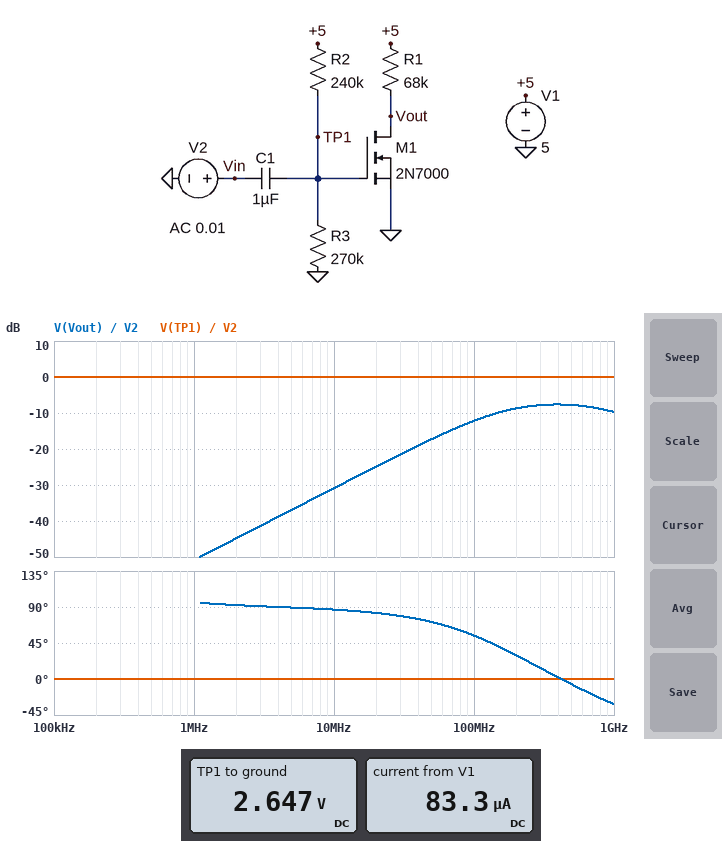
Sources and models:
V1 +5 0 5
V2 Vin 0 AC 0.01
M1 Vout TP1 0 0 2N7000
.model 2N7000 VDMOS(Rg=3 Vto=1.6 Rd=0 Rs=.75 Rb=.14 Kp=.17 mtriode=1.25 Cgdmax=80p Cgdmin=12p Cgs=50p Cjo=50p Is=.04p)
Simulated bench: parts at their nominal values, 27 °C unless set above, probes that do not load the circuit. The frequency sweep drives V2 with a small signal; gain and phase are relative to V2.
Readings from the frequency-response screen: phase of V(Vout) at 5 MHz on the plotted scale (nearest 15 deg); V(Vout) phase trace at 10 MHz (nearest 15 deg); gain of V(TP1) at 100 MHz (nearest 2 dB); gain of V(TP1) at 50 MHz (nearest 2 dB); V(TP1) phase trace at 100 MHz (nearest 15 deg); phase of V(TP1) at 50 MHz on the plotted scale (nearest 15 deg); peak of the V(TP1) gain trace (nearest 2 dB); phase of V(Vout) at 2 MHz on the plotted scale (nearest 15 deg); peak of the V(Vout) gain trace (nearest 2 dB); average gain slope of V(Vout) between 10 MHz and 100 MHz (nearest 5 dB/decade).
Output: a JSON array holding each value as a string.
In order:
["90 deg", "90 deg", "0 dB", "0 dB", "0 deg", "0 deg", "0 dB", "90 deg", "-8 dB", "20 dB/decade"]
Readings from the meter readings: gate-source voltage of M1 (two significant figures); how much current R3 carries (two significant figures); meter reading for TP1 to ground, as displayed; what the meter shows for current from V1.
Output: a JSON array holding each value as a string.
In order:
["2.6 V", "9.8 µA", "2.647 V", "83.3 µA"]
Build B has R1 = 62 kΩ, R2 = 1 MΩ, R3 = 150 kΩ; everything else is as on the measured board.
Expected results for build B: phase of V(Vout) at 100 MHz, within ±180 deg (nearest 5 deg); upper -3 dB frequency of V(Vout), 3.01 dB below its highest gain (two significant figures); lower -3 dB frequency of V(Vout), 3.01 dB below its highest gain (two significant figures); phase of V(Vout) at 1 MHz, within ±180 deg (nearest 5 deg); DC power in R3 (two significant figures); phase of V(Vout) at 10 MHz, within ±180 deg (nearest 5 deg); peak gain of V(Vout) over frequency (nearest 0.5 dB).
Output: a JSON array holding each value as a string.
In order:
["-5 deg", "780 MHz", "70 kHz", "5 deg", "2.8 µW", "0 deg", "-6.0 dB"]
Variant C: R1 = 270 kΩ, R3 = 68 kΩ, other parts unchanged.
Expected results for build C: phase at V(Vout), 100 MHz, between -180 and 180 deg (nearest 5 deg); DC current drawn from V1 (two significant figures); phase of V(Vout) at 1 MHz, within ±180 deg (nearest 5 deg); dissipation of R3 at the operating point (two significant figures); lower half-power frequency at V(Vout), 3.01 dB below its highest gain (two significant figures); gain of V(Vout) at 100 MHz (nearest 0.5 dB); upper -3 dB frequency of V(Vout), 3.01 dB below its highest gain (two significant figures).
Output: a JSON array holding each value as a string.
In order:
["-5 deg", "16 µA", "0 deg", "18 µW", "12 kHz", "-6.0 dB", "780 MHz"]
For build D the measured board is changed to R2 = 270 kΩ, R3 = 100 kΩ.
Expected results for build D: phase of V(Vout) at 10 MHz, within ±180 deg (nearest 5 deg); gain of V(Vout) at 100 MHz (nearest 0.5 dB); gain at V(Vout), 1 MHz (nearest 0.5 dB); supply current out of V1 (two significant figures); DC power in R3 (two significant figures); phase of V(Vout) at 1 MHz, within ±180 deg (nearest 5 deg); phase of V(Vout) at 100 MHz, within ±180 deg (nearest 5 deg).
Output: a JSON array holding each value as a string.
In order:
["5 deg", "-6.0 dB", "-3.5 dB", "19 µA", "18 µW", "45 deg", "-5 deg"]
